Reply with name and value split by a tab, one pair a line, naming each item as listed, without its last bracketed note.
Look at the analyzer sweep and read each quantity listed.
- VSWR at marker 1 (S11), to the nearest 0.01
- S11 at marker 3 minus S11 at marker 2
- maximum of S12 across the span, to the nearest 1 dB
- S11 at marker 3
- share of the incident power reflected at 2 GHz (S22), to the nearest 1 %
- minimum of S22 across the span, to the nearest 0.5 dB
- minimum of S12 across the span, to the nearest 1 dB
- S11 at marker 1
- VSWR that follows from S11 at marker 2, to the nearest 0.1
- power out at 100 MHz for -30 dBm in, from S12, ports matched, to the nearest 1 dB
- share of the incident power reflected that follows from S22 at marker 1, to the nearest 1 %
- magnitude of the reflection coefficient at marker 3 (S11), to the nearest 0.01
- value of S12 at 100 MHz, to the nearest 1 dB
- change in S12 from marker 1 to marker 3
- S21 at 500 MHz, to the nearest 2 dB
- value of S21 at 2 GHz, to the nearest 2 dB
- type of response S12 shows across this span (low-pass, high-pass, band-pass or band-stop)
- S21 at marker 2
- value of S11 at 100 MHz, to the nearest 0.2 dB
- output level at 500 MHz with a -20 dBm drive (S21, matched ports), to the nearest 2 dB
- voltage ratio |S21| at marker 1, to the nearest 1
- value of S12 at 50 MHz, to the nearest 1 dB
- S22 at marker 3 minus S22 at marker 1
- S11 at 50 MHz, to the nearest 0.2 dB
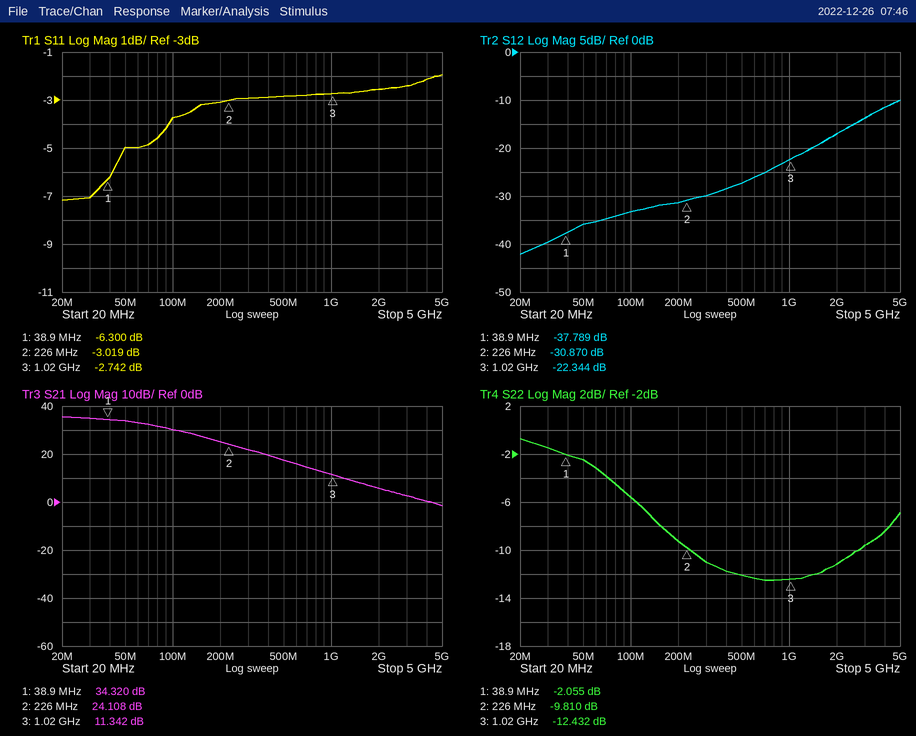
VSWR at marker 1 (S11), to the nearest 0.01	2.88
S11 at marker 3 minus S11 at marker 2	0.277 dB
maximum of S12 across the span, to the nearest 1 dB	-10 dB
S11 at marker 3	-2.742 dB
share of the incident power reflected at 2 GHz (S22), to the nearest 1 %	8 %
minimum of S22 across the span, to the nearest 0.5 dB	-12.5 dB
minimum of S12 across the span, to the nearest 1 dB	-42 dB
S11 at marker 1	-6.300 dB
VSWR that follows from S11 at marker 2, to the nearest 0.1	5.8
power out at 100 MHz for -30 dBm in, from S12, ports matched, to the nearest 1 dB	-63 dBm
share of the incident power reflected that follows from S22 at marker 1, to the nearest 1 %	62 %
magnitude of the reflection coefficient at marker 3 (S11), to the nearest 0.01	0.73
value of S12 at 100 MHz, to the nearest 1 dB	-33 dB
change in S12 from marker 1 to marker 3	15.445 dB
S21 at 500 MHz, to the nearest 2 dB	18 dB
value of S21 at 2 GHz, to the nearest 2 dB	6 dB
type of response S12 shows across this span	high-pass
S21 at marker 2	24.108 dB
value of S11 at 100 MHz, to the nearest 0.2 dB	-3.8 dB
output level at 500 MHz with a -20 dBm drive (S21, matched ports), to the nearest 2 dB	-2 dBm
voltage ratio |S21| at marker 1, to the nearest 1	52
value of S12 at 50 MHz, to the nearest 1 dB	-36 dB
S22 at marker 3 minus S22 at marker 1	-10.377 dB
S11 at 50 MHz, to the nearest 0.2 dB	-5.0 dB
